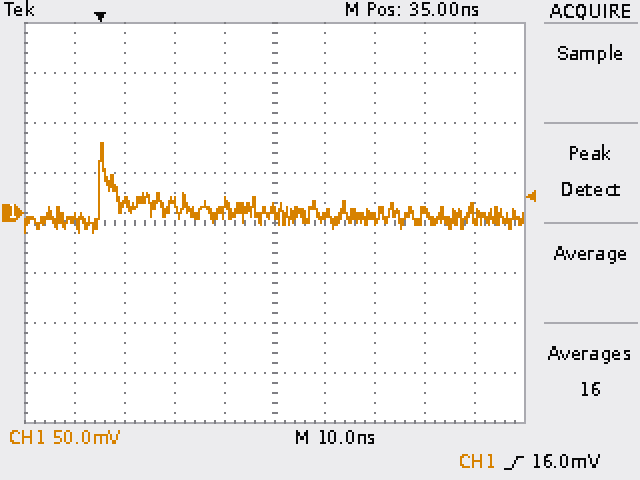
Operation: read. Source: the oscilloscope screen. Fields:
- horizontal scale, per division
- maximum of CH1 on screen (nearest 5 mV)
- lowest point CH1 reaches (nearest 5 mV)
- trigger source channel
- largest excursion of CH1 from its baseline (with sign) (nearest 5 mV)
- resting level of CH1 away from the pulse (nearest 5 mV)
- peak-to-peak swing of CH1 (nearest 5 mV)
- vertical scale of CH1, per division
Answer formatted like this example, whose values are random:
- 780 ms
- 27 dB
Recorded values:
- 10 ns
- 70 mV
- -20 mV
- CH1
- +75 mV
- -5 mV
- 90 mV
- 50 mV
